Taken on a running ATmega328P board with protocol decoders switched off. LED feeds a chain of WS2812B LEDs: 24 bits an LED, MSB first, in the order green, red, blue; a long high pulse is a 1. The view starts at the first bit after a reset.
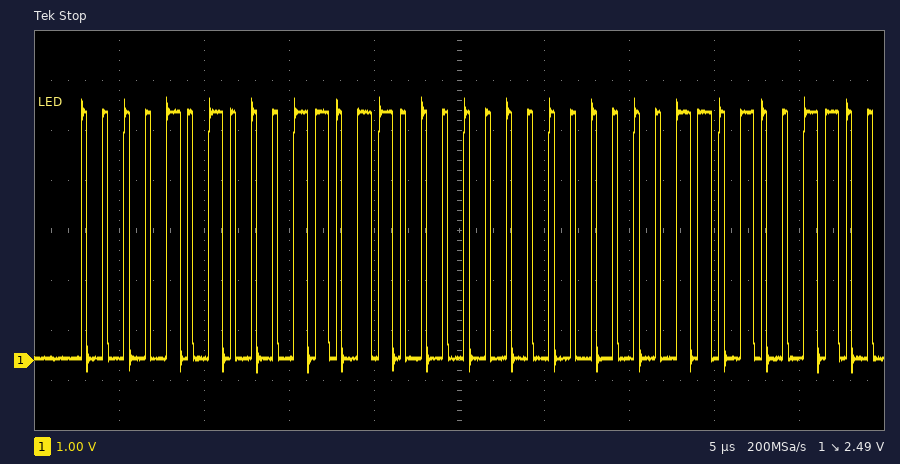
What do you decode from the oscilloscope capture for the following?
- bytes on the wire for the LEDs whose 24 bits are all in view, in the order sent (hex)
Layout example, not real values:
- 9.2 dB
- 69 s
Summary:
- 0A 36 00
